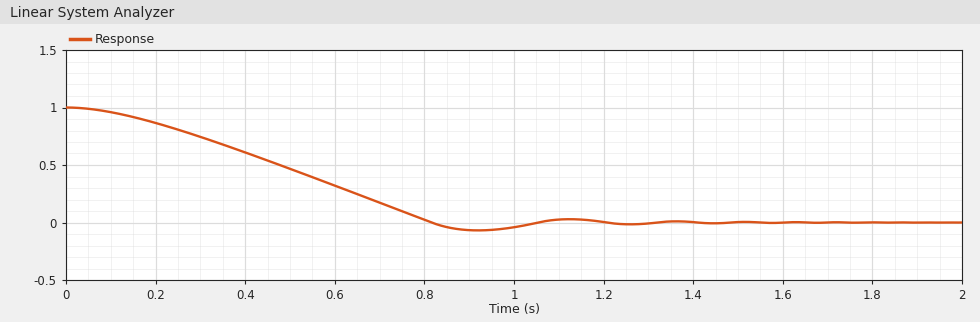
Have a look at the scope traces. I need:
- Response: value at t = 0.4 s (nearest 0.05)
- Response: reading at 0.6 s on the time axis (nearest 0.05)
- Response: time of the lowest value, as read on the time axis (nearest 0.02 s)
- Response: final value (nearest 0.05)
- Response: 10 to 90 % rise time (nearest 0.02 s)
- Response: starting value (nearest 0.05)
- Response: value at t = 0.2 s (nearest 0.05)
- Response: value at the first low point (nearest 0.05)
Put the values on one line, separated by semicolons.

0.60; 0.30; 0.92 s; 0.00; 0.58 s; 1.00; 0.85; -0.05
